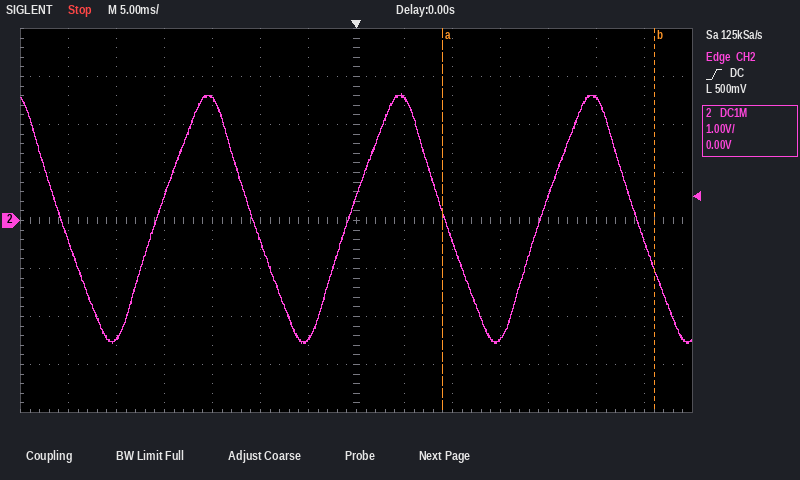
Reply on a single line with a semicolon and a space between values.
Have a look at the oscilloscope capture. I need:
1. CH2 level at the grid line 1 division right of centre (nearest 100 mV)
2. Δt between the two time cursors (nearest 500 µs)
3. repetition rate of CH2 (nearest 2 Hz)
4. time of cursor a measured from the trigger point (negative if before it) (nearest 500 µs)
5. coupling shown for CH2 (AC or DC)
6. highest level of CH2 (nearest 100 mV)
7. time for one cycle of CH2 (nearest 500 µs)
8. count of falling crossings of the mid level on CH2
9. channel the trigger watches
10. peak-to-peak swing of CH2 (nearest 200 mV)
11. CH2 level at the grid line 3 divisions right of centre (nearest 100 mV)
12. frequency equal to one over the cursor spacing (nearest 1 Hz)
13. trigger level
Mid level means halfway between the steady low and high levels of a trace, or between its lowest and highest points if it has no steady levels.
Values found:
2.5 V; 22.0 ms; 50 Hz; +9.0 ms; DC; 2.6 V; 20.0 ms; 4; CH2; 5.2 V; -2.5 V; 45 Hz; 500 mV
